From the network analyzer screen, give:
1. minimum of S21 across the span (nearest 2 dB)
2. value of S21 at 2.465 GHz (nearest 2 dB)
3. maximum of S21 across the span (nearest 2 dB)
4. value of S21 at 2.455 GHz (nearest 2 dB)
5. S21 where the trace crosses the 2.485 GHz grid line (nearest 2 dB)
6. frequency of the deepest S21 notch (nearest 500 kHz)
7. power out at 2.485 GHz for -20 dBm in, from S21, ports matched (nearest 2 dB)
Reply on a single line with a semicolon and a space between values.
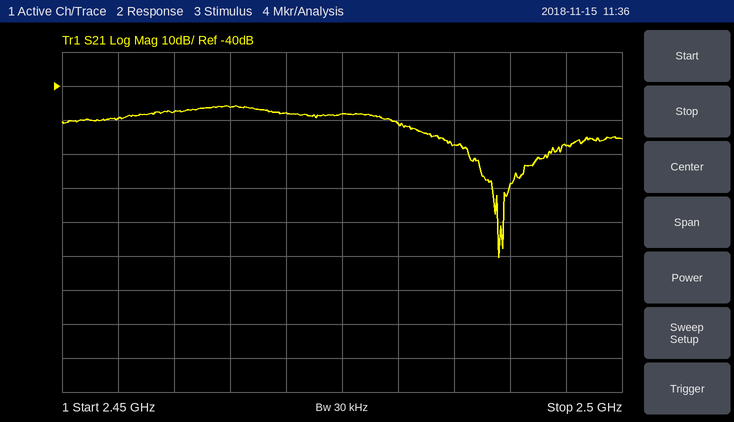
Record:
-90 dB; -46 dB; -46 dB; -50 dB; -58 dB; 2.4890 GHz; -78 dBm
